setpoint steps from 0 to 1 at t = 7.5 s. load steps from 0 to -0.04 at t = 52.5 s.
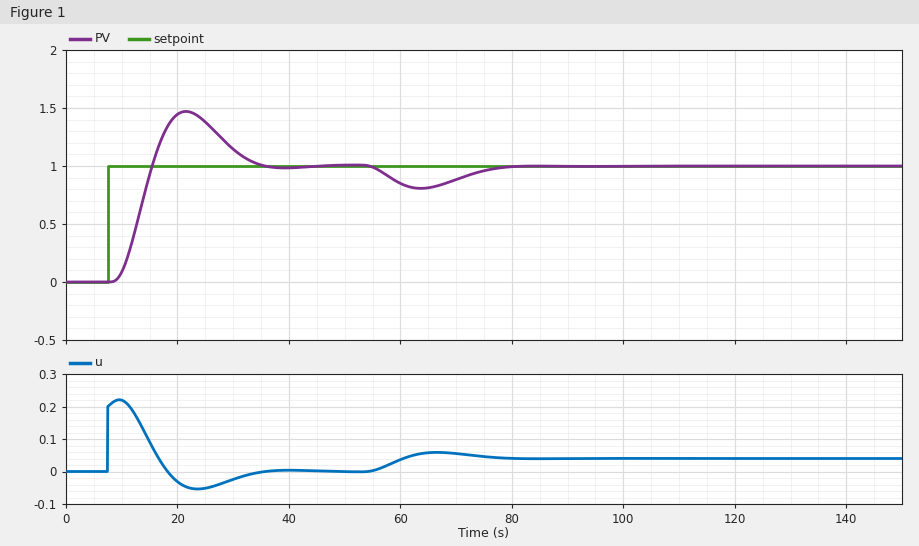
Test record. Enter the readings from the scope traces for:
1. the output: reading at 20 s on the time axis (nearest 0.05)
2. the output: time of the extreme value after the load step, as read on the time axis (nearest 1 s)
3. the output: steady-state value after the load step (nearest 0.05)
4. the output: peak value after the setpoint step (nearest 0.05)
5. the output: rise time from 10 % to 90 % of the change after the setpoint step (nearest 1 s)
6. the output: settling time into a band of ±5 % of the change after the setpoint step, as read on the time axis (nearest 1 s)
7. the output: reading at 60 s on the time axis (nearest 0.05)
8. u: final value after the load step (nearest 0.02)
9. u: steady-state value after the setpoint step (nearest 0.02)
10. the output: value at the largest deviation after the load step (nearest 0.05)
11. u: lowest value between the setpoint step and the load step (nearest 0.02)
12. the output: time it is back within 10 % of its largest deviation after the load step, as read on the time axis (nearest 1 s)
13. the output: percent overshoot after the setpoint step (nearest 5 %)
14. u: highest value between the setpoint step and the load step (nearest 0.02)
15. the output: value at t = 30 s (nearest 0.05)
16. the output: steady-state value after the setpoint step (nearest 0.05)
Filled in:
1.45
64 s
1.00
1.45
5 s
33 s
0.85
0.04
0.00
0.80
-0.06
77 s
45 %
0.22
1.15
1.00
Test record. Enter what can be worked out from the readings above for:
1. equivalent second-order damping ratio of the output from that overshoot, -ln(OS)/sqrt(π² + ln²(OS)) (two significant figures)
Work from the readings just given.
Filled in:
0.25
